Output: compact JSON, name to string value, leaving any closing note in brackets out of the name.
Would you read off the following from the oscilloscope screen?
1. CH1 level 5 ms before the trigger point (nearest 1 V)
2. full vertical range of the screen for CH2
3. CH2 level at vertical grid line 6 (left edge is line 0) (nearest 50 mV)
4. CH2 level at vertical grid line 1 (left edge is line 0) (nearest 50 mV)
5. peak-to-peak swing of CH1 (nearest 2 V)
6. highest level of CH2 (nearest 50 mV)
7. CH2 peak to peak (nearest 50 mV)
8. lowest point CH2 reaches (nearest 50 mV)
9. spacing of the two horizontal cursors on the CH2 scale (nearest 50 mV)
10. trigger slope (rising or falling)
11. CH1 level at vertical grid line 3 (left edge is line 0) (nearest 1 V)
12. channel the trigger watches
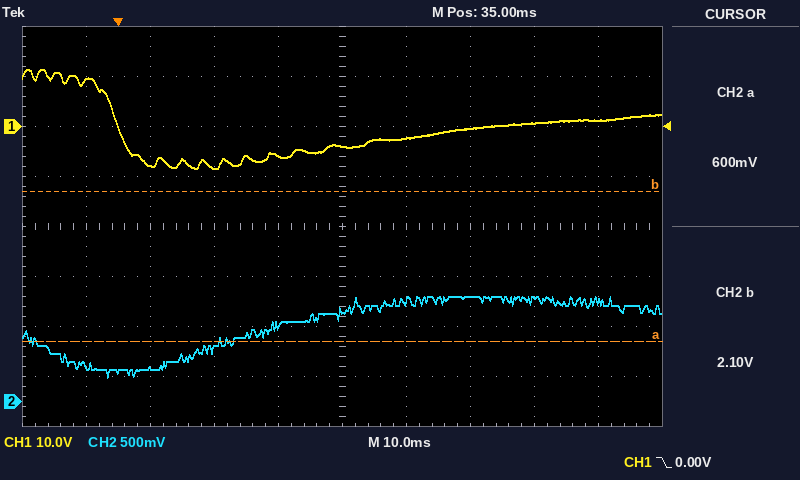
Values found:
{"CH1 level 5 ms before the trigger point": "9 V", "full vertical range of the screen for CH2": "4 V", "CH2 level at vertical grid line 6 (left edge is line 0)": "1.00 V", "CH2 level at vertical grid line 1 (left edge is line 0)": "350 mV", "peak-to-peak swing of CH1": "20 V", "highest level of CH2": "1.05 V", "CH2 peak to peak": "800 mV", "lowest point CH2 reaches": "250 mV", "spacing of the two horizontal cursors on the CH2 scale": "1.50 V", "trigger slope": "falling", "CH1 level at vertical grid line 3 (left edge is line 0)": "-8 V", "channel the trigger watches": "CH1"}
